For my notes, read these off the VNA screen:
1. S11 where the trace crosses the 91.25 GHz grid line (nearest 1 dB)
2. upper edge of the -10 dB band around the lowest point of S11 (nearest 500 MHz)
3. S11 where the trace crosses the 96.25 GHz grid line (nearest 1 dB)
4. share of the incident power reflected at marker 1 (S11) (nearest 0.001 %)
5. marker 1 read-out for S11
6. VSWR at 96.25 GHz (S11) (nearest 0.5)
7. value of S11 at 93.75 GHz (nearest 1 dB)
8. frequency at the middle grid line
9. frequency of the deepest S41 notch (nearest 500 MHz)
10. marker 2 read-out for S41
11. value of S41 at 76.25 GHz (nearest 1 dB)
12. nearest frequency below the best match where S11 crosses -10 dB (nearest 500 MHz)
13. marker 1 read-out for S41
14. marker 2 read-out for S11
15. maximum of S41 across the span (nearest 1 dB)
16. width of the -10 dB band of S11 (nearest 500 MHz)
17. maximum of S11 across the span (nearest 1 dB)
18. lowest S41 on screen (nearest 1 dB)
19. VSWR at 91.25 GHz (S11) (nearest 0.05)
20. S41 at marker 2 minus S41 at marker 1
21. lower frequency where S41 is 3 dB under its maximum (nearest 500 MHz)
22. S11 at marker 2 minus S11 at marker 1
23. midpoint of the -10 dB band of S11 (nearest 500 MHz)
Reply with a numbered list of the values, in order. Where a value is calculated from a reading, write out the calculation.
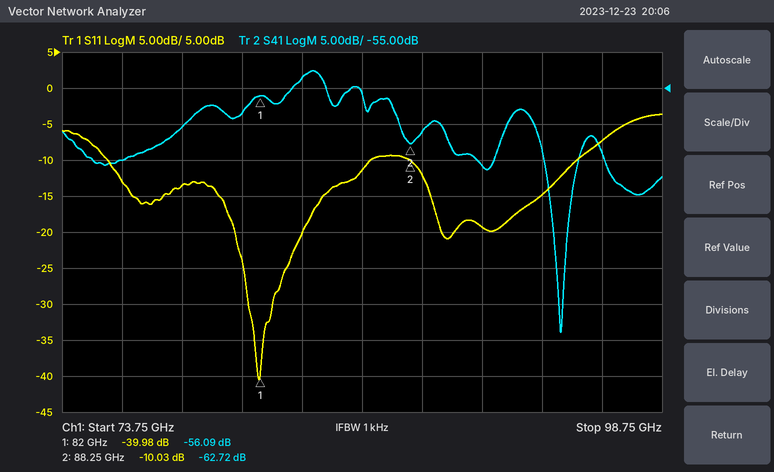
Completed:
1. -19 dB
2. 86.5 GHz
3. -7 dB
4. 10^(-39.98/10) ≈ 0.010 %
5. -39.98 dB
6. |Γ| = 10^(-7/20) = 0.4467; VSWR = (1 + 0.4467)/(1 − 0.4467) ≈ 2.61, so 2.5 to the nearest 0.5
7. -15 dB
8. 86.25 GHz
9. 94.5 GHz
10. -62.72 dB
11. -65 dB
12. 75.5 GHz
13. -56.09 dB
14. -10.03 dB
15. -53 dB
16. 86.5 GHz − 75.5 GHz = 11.0 GHz
17. -4 dB
18. -89 dB
19. |Γ| = 10^(-19/20) = 0.1122; VSWR = (1 + 0.1122)/(1 − 0.1122) ≈ 1.25
20. -62.72 − (-56.09) = -6.63 dB
21. 83.0 GHz
22. -10.03 − (-39.98) = 29.95 dB
23. 81.0 GHz
